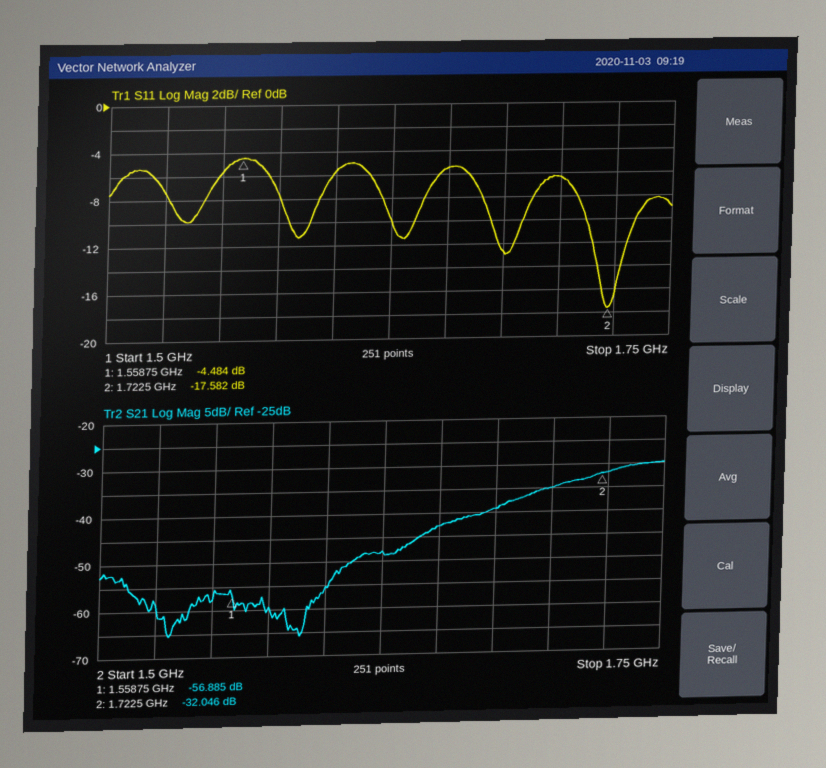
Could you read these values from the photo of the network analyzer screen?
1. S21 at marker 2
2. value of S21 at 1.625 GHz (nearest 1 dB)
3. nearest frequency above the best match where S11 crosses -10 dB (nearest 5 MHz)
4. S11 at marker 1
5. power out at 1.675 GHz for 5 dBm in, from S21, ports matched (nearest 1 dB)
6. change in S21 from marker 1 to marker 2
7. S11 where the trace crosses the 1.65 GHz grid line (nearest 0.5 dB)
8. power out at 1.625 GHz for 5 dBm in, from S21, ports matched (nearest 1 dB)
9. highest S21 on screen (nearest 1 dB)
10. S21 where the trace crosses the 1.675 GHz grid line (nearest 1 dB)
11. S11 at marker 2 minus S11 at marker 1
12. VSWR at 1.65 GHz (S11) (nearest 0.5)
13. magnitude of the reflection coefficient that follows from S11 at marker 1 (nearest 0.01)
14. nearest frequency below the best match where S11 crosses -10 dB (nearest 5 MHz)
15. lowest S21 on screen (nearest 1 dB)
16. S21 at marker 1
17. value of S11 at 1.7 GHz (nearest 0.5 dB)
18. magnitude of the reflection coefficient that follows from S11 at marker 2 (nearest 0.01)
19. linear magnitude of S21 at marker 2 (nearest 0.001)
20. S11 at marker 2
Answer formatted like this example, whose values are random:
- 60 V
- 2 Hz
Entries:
- -32.046 dB
- -48 dB
- 1.735 GHz
- -4.484 dB
- -34 dBm
- 24.839 dB
- -5.5 dB
- -43 dBm
- -30 dB
- -39 dB
- -13.098 dB
- 3.5
- 0.60
- 1.710 GHz
- -66 dB
- -56.885 dB
- -6.5 dB
- 0.13
- 0.025
- -17.582 dB
